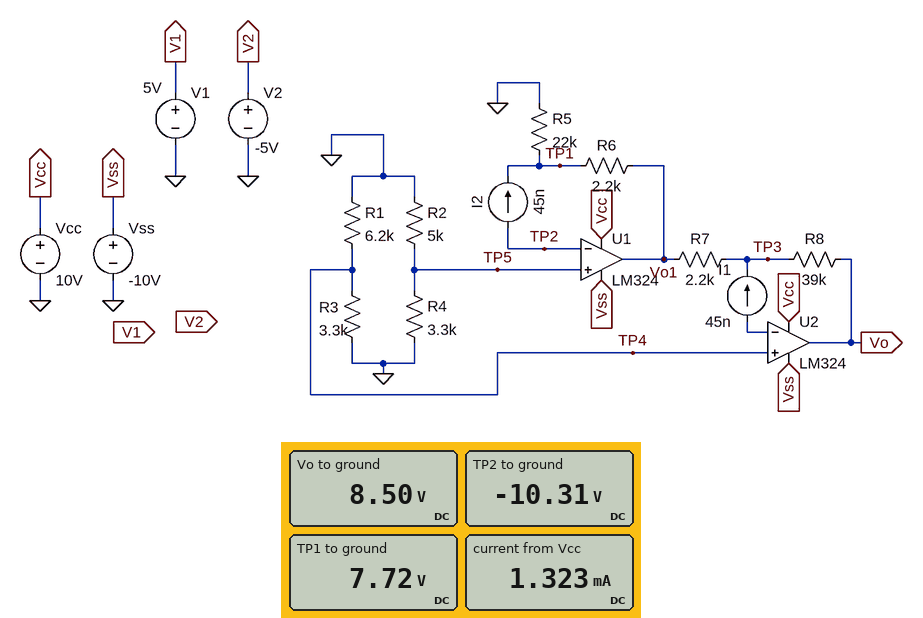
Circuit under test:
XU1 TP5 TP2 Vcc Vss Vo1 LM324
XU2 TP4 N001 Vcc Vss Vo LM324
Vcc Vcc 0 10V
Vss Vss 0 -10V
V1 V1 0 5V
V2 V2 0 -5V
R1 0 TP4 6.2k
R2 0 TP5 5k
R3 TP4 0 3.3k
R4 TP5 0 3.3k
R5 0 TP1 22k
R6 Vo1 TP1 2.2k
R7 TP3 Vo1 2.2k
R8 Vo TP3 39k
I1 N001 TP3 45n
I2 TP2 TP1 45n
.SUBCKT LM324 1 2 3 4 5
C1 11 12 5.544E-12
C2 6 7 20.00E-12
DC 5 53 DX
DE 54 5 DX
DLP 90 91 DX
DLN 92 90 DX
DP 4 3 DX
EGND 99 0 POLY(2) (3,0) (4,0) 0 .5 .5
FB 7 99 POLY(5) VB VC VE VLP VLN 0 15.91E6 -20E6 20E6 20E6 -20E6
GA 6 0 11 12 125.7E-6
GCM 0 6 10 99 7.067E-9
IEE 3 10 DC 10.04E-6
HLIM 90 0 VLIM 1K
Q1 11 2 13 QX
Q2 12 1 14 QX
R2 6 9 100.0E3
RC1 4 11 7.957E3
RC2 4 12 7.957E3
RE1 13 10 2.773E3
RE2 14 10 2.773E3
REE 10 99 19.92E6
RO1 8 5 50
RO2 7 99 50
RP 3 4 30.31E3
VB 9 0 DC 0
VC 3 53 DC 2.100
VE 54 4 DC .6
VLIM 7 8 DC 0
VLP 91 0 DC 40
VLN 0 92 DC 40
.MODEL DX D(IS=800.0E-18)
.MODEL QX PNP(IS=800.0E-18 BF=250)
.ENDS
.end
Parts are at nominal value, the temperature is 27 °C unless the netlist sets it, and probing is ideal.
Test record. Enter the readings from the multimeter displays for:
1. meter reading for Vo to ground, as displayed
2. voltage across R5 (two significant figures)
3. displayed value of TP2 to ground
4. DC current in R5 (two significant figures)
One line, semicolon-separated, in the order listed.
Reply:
8.50 V; 7.7 V; -10.31 V; 350 µA
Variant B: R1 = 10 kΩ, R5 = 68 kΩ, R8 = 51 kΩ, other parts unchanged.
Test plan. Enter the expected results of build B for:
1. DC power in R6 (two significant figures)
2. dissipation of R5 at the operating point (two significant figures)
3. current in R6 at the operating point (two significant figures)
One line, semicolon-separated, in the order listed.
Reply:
32 µW; 1.0 mW; 120 µA
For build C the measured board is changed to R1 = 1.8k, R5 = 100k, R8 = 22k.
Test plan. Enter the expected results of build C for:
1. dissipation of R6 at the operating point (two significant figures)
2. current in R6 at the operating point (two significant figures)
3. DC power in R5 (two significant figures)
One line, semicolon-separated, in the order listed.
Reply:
15 µW; 83 µA; 690 µW
